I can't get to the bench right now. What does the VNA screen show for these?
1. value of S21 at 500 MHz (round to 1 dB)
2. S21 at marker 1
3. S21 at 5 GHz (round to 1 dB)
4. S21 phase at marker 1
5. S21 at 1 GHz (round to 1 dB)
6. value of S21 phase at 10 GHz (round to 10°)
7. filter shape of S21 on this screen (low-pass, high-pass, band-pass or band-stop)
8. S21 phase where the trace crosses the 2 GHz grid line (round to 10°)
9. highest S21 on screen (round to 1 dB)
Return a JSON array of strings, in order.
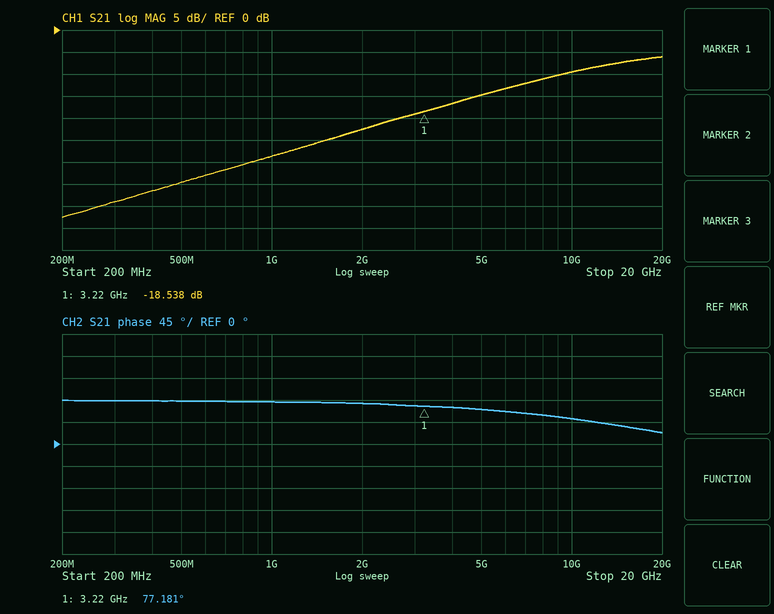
["-35 dB", "-18.538 dB", "-15 dB", "77.181°", "-29 dB", "50°", "high-pass", "80°", "-6 dB"]
